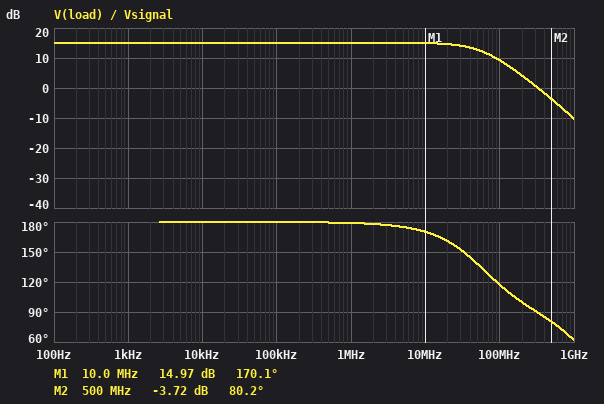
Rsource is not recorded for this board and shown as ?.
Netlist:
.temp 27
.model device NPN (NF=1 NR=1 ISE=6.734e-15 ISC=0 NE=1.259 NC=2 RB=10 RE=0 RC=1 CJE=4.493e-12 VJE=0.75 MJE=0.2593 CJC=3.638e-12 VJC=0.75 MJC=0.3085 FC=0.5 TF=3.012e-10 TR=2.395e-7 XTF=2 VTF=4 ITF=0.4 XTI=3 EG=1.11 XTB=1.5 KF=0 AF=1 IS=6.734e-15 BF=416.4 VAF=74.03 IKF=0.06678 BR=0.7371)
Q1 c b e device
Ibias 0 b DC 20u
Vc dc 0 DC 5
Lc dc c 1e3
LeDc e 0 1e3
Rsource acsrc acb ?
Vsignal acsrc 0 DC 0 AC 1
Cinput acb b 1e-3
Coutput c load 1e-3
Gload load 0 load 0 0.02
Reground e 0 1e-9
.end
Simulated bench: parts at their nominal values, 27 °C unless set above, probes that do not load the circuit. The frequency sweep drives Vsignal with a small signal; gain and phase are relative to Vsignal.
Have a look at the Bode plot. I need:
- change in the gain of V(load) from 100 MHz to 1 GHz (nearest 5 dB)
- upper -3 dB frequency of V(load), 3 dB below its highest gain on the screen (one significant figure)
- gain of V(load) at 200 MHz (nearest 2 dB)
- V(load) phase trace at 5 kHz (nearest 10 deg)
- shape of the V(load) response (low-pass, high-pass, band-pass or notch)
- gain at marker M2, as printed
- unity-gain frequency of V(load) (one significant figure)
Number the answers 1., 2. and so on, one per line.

1. -20 dB
2. 60 MHz
3. 4 dB
4. 180 deg
5. low-pass
6. -3.72 dB
7. 300 MHz
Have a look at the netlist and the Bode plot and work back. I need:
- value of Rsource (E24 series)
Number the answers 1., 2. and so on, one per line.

1. 39 Ω
